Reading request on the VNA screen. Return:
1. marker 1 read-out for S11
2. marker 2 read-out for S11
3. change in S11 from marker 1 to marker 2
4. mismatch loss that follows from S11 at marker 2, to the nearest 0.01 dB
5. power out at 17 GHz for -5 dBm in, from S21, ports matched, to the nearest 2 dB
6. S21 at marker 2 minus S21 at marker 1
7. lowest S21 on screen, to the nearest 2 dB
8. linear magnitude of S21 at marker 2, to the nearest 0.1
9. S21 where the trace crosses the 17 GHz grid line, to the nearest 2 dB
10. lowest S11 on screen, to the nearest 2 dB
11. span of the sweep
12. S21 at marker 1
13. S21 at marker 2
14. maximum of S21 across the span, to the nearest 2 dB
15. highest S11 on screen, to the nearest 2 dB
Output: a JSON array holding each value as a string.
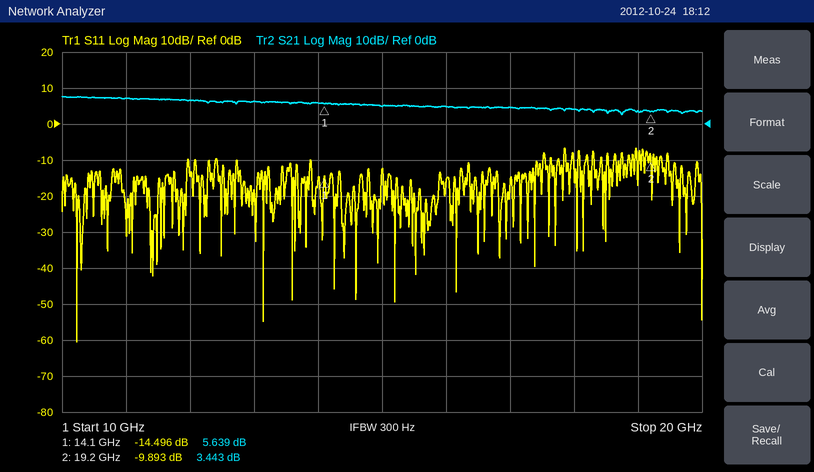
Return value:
["-14.496 dB", "-9.893 dB", "4.603 dB", "0.47 dB", "0 dBm", "-2.196 dB", "2 dB", "1.5", "4 dB", "-60 dB", "10 GHz", "5.639 dB", "3.443 dB", "8 dB", "-6 dB"]
